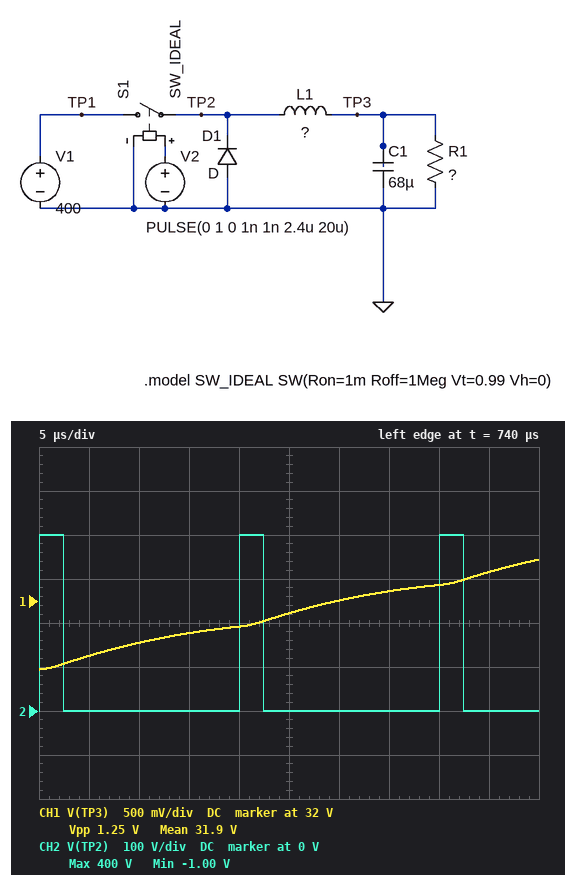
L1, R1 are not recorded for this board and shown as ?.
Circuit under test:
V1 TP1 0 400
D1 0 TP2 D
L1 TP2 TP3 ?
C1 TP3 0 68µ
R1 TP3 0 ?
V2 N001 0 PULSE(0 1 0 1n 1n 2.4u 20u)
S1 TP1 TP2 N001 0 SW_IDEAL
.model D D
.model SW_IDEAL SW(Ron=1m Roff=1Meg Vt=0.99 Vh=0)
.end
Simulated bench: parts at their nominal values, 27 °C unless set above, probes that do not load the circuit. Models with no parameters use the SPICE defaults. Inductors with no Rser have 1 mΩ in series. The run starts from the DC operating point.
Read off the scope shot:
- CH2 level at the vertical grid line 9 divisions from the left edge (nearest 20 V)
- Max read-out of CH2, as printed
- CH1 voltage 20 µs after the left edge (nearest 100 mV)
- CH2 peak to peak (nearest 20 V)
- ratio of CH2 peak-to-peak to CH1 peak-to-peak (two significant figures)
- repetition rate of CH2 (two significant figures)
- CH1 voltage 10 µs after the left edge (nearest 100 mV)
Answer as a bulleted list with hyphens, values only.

- 0 V
- 400 V
- 31.7 V
- 400 V
- 320
- 50 kHz
- 31.5 V
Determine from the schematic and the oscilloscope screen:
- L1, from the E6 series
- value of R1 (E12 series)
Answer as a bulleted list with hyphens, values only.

- 470 µH
- 0.68 Ω
